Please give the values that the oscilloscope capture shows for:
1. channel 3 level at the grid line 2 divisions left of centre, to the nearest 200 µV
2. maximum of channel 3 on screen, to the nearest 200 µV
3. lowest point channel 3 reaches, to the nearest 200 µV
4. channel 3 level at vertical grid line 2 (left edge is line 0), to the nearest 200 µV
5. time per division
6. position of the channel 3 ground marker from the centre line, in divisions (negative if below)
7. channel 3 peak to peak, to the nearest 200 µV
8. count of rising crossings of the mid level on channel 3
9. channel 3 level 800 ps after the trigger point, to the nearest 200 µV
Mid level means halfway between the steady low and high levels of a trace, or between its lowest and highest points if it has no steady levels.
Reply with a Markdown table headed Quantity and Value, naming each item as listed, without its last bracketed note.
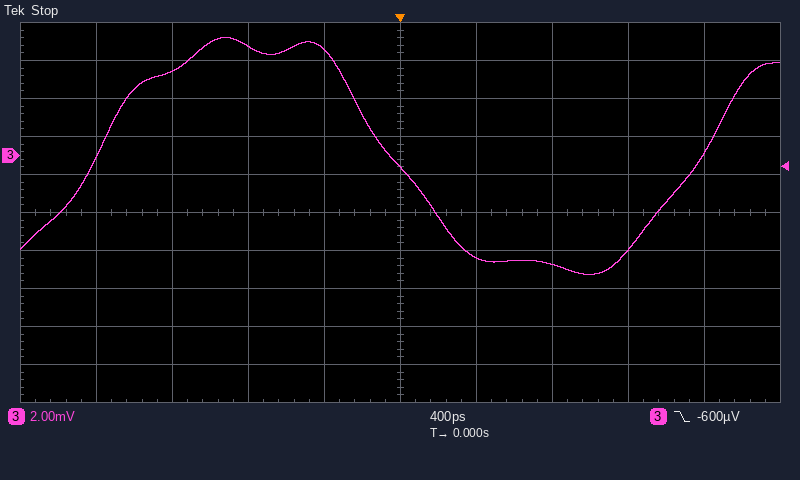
| Quantity | Value |
|---|---|
| channel 3 level at the grid line 2 divisions left of centre, to the nearest 200 µV | 5.8 mV |
| maximum of channel 3 on screen, to the nearest 200 µV | 6.2 mV |
| lowest point channel 3 reaches, to the nearest 200 µV | -6.2 mV |
| channel 3 level at vertical grid line 2 (left edge is line 0), to the nearest 200 µV | 4.4 mV |
| time per division | 400 ps |
| position of the channel 3 ground marker from the centre line, in divisions | +1.5 div |
| channel 3 peak to peak, to the nearest 200 µV | 12.4 mV |
| count of rising crossings of the mid level on channel 3 | 2 |
| channel 3 level 800 ps after the trigger point, to the nearest 200 µV | -5.8 mV |
